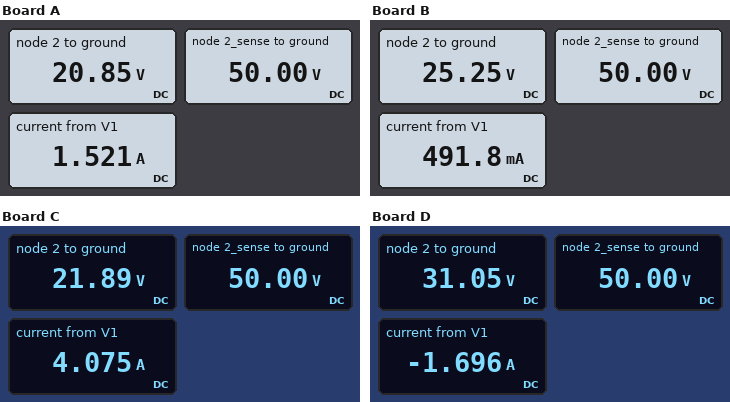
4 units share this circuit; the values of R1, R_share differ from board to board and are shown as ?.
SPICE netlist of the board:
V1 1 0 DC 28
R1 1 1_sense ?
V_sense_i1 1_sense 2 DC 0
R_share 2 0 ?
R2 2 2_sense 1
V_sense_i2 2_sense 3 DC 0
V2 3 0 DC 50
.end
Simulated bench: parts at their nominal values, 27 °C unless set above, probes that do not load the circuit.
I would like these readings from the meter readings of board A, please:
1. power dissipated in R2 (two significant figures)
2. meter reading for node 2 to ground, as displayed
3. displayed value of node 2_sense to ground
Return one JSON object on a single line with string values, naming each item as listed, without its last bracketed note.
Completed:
{"power dissipated in R2": "850 W", "meter reading for node 2 to ground, as displayed": "20.85 V", "displayed value of node 2_sense to ground": "50.00 V"}
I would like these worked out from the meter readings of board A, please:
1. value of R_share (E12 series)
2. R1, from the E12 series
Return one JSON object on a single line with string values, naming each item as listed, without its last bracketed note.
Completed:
{"value of R_share": "0.68 Ω", "R1, from the E12 series": "4.7 Ω"}
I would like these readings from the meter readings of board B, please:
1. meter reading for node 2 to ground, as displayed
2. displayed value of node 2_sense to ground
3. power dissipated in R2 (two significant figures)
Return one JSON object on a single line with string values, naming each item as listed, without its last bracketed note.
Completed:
{"meter reading for node 2 to ground, as displayed": "25.25 V", "displayed value of node 2_sense to ground": "50.00 V", "power dissipated in R2": "610 W"}
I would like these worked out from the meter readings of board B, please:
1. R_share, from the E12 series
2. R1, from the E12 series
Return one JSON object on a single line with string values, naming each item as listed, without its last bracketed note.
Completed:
{"R_share, from the E12 series": "1 Ω", "R1, from the E12 series": "5.6 Ω"}
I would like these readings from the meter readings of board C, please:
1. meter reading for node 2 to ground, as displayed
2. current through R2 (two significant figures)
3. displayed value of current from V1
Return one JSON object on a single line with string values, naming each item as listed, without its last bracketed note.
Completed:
{"meter reading for node 2 to ground, as displayed": "21.89 V", "current through R2": "28 A", "displayed value of current from V1": "4.075 A"}
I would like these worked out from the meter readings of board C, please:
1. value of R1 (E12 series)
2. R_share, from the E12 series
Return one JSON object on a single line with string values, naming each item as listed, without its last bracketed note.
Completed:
{"value of R1": "1.5 Ω", "R_share, from the E12 series": "0.68 Ω"}
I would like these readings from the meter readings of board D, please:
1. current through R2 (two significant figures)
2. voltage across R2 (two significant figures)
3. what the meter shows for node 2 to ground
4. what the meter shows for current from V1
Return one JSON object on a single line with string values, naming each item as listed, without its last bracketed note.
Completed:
{"current through R2": "19 A", "voltage across R2": "19 V", "what the meter shows for node 2 to ground": "31.05 V", "what the meter shows for current from V1": "-1.696 A"}
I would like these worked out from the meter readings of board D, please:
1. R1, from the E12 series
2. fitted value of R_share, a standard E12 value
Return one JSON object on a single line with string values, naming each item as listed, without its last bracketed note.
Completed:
{"R1, from the E12 series": "1.8 Ω", "fitted value of R_share, a standard E12 value": "1.8 Ω"}
